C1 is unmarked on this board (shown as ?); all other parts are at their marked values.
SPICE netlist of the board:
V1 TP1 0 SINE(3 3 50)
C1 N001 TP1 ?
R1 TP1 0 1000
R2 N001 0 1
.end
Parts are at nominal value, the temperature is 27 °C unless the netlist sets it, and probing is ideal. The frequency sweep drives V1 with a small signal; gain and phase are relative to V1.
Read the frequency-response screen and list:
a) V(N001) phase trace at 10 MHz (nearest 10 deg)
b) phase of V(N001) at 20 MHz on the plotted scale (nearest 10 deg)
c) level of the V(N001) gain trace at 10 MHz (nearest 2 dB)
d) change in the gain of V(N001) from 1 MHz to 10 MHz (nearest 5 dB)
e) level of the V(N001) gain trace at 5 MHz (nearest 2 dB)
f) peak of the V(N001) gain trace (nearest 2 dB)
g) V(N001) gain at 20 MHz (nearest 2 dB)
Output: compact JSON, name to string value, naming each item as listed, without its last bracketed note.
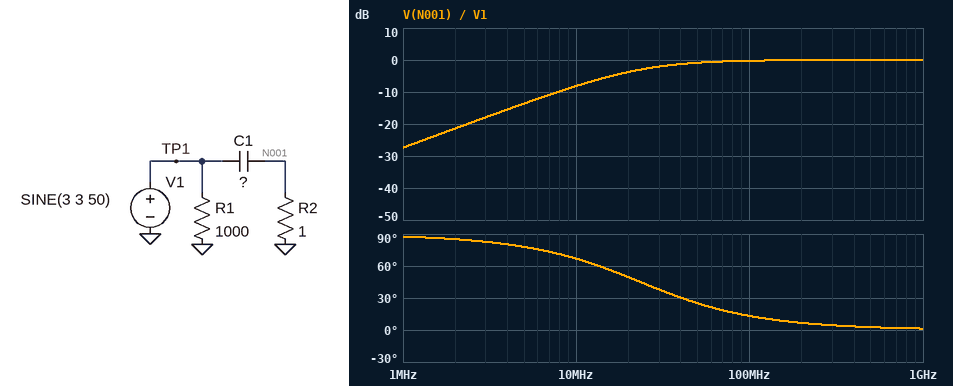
{"V(N001) phase trace at 10 MHz": "70 deg", "phase of V(N001) at 20 MHz on the plotted scale": "50 deg", "level of the V(N001) gain trace at 10 MHz": "-8 dB", "change in the gain of V(N001) from 1 MHz to 10 MHz": "20 dB", "level of the V(N001) gain trace at 5 MHz": "-14 dB", "peak of the V(N001) gain trace": "0 dB", "V(N001) gain at 20 MHz": "-4 dB"}
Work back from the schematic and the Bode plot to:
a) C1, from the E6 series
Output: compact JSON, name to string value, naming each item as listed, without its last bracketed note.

{"C1, from the E6 series": "6.8 nF"}
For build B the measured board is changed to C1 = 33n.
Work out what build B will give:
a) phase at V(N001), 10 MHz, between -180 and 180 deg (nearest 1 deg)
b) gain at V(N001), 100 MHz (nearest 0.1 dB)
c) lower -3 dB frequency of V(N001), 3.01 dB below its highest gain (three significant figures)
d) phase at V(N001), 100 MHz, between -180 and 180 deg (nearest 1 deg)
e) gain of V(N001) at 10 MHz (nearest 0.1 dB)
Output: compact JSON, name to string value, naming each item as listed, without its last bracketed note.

{"phase at V(N001), 10 MHz, between -180 and 180 deg": "26 deg", "gain at V(N001), 100 MHz": "0 dB", "lower -3 dB frequency of V(N001), 3.01 dB below its highest gain": "4.82 MHz", "phase at V(N001), 100 MHz, between -180 and 180 deg": "3 deg", "gain of V(N001) at 10 MHz": "-0.9 dB"}
